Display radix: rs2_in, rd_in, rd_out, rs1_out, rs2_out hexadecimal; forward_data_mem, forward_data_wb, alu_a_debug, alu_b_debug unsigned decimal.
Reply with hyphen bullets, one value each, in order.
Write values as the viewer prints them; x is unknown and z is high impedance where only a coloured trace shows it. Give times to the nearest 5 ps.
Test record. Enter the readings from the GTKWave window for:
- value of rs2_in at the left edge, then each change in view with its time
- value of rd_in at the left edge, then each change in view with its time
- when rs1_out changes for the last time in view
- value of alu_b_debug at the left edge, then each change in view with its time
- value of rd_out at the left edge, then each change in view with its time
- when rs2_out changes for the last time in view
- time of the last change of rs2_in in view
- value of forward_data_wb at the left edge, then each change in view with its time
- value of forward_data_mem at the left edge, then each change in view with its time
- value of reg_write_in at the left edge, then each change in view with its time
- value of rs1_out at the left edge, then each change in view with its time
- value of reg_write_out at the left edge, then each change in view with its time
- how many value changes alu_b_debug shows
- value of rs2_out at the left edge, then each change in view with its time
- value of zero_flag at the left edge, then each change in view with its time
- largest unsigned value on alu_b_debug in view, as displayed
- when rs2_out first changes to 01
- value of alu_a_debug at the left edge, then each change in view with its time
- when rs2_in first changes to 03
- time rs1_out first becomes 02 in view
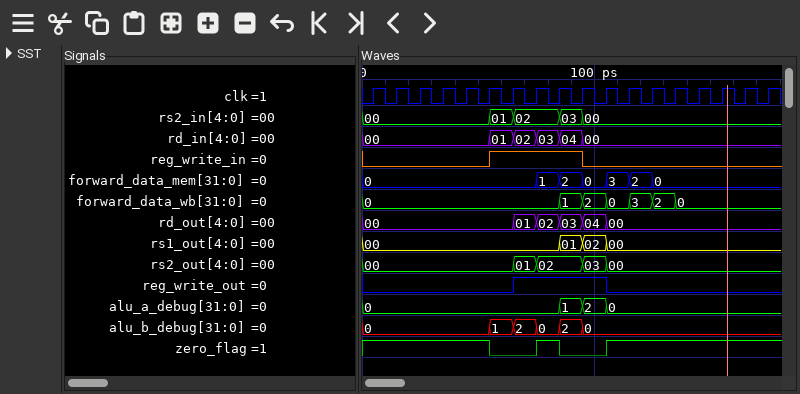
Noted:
- 00, 01 at 55 ps, 02 at 65 ps, 03 at 85 ps, 00 at 95 ps
- 00, 01 at 55 ps, 02 at 65 ps, 03 at 75 ps, 04 at 85 ps, 00 at 95 ps
- 105 ps
- 0, 1 at 55 ps, 2 at 65 ps, 0 at 75 ps, 2 at 85 ps, 0 at 95 ps
- 00, 01 at 65 ps, 02 at 75 ps, 03 at 85 ps, 04 at 95 ps, 00 at 105 ps
- 105 ps
- 95 ps
- 0, 1 at 85 ps, 2 at 95 ps, 0 at 105 ps, 3 at 115 ps, 2 at 125 ps, 0 at 135 ps
- 0, 1 at 75 ps, 2 at 85 ps, 0 at 95 ps, 3 at 105 ps, 2 at 115 ps, 0 at 125 ps
- 0, 1 at 55 ps, 0 at 95 ps
- 00, 01 at 85 ps, 02 at 95 ps, 00 at 105 ps
- 0, 1 at 65 ps, 0 at 105 ps
- 5
- 00, 01 at 65 ps, 02 at 75 ps, 03 at 95 ps, 00 at 105 ps
- 1, 0 at 55 ps, 1 at 75 ps, 0 at 85 ps, 1 at 105 ps
- 2
- 65 ps
- 0, 1 at 85 ps, 2 at 95 ps, 0 at 105 ps
- 85 ps
- 95 ps
